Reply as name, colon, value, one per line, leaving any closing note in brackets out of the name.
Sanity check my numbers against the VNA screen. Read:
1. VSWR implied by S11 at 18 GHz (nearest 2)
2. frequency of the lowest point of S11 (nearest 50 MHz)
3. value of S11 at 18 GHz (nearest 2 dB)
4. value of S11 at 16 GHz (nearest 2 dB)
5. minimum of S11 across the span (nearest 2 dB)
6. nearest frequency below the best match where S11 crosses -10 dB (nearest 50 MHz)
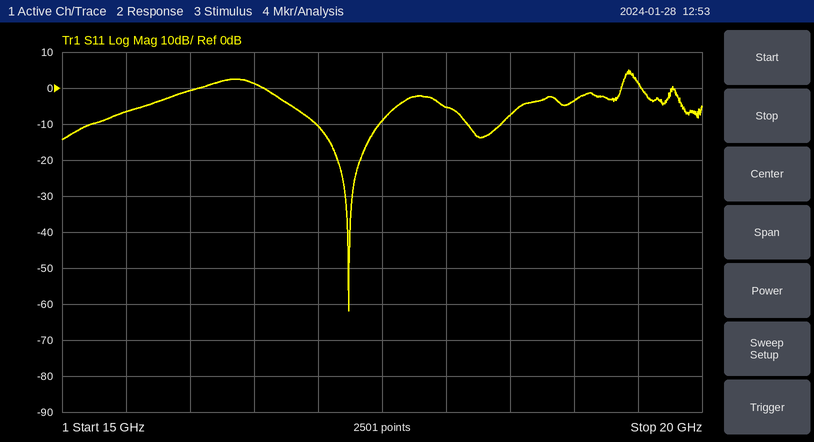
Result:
VSWR implied by S11 at 18 GHz: 4
frequency of the lowest point of S11: 17.25 GHz
value of S11 at 18 GHz: -6 dB
value of S11 at 16 GHz: 0 dB
minimum of S11 across the span: -62 dB
nearest frequency below the best match where S11 crosses -10 dB: 17.00 GHz
